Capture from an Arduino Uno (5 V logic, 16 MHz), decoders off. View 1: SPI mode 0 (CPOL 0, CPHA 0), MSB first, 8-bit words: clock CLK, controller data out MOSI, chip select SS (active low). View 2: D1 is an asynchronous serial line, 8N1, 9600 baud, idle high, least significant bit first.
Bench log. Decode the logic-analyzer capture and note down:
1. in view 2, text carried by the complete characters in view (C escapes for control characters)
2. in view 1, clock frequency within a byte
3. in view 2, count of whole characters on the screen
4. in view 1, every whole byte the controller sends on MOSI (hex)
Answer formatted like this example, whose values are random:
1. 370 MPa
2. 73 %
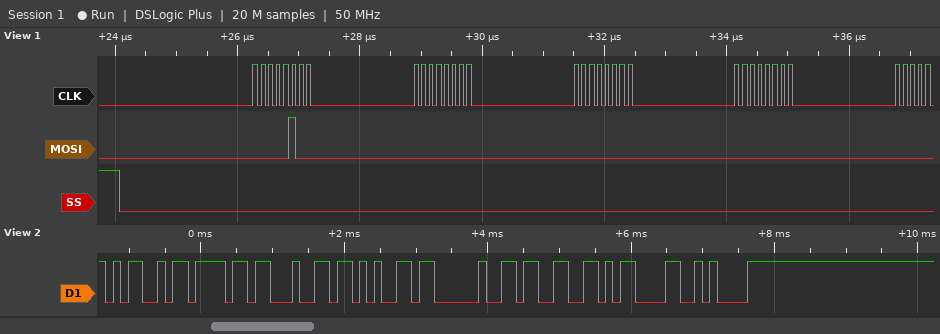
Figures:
1. "Mode 3\r\n"
2. 8 MHz
3. 8
4. 04 00 00 00
